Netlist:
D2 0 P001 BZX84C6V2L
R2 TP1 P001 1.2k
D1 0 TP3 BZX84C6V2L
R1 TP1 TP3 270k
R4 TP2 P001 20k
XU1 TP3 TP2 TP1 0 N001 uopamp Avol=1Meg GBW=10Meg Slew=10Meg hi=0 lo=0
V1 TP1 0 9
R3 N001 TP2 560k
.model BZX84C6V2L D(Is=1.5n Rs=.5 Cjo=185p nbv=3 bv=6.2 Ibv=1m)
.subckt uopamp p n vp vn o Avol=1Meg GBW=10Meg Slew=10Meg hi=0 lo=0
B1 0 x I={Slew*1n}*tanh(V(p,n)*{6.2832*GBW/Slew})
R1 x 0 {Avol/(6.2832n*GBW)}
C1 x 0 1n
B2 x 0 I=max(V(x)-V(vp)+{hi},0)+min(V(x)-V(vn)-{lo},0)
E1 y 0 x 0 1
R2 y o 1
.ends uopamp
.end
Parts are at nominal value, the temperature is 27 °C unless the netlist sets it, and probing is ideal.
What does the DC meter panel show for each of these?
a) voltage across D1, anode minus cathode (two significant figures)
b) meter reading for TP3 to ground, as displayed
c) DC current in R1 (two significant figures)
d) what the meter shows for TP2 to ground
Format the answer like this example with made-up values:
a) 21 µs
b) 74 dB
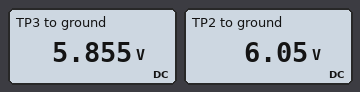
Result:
a) -5.9 V
b) 5.855 V
c) 12 µA
d) 6.05 V
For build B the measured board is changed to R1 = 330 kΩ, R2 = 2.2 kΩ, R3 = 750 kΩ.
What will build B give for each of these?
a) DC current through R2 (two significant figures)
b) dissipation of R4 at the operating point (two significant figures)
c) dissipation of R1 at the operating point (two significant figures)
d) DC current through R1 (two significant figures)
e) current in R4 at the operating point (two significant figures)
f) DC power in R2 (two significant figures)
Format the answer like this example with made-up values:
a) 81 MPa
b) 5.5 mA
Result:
a) 1.3 mA
b) 1.3 µW
c) 30 µW
d) 9.6 µA
e) 8.1 µA
f) 3.5 mW
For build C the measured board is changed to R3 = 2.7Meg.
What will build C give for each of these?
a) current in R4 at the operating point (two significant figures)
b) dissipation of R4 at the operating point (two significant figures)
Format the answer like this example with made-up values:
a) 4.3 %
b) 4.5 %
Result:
a) 2.3 µA
b) 110 nW
